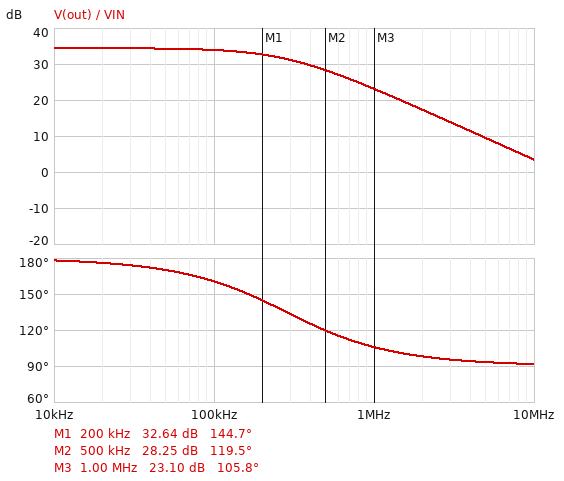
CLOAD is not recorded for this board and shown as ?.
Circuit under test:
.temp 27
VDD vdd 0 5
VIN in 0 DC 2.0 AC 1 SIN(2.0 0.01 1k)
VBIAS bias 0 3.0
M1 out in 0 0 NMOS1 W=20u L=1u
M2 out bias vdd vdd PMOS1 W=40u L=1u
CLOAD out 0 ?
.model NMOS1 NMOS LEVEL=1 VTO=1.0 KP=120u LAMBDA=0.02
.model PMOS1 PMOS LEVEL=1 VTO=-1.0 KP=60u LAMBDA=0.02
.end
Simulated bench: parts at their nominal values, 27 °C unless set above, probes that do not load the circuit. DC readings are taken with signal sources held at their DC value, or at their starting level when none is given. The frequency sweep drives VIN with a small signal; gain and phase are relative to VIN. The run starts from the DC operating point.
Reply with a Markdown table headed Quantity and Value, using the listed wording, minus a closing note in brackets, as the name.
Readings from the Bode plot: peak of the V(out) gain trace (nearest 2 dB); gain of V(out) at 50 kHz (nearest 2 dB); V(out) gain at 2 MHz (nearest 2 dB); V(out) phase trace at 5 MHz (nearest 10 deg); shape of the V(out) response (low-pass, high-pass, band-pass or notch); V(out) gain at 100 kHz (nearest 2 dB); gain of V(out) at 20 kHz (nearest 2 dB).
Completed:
| Quantity | Value |
|---|---|
| peak of the V(out) gain trace | 34 dB |
| gain of V(out) at 50 kHz | 34 dB |
| V(out) gain at 2 MHz | 18 dB |
| V(out) phase trace at 5 MHz | 90 deg |
| shape of the V(out) response | low-pass |
| V(out) gain at 100 kHz | 34 dB |
| gain of V(out) at 20 kHz | 34 dB |
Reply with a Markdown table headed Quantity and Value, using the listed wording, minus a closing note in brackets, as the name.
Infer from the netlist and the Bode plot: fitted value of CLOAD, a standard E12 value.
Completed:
| Quantity | Value |
|---|---|
| fitted value of CLOAD, a standard E12 value | 27 pF |
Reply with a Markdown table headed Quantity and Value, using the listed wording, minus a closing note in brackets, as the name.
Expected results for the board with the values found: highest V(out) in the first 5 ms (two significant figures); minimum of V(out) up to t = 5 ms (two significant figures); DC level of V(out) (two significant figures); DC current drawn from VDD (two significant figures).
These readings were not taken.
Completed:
| Quantity | Value |
|---|---|
| highest V(out) in the first 5 ms | 3.0 V |
| minimum of V(out) up to t = 5 ms | 2.0 V |
| DC level of V(out) | 2.5 V |
| DC current drawn from VDD | 1.3 mA |
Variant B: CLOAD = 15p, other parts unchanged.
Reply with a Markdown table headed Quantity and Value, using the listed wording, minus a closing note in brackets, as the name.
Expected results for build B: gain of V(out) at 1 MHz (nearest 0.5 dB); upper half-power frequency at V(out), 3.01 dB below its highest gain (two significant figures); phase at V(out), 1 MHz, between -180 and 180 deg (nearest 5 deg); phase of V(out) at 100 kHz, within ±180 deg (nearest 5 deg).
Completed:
| Quantity | Value |
|---|---|
| gain of V(out) at 1 MHz | 27.5 dB |
| upper half-power frequency at V(out), 3.01 dB below its highest gain | 510 kHz |
| phase at V(out), 1 MHz, between -180 and 180 deg | 115 deg |
| phase of V(out) at 100 kHz, within ±180 deg | 170 deg |
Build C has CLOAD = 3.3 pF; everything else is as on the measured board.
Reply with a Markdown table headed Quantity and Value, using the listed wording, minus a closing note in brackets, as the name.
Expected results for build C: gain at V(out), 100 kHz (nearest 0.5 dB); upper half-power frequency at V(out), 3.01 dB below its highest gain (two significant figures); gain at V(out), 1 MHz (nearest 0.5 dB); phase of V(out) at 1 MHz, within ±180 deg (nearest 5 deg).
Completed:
| Quantity | Value |
|---|---|
| gain at V(out), 100 kHz | 34.5 dB |
| upper half-power frequency at V(out), 3.01 dB below its highest gain | 2.3 MHz |
| gain at V(out), 1 MHz | 33.5 dB |
| phase of V(out) at 1 MHz, within ±180 deg | 155 deg |
